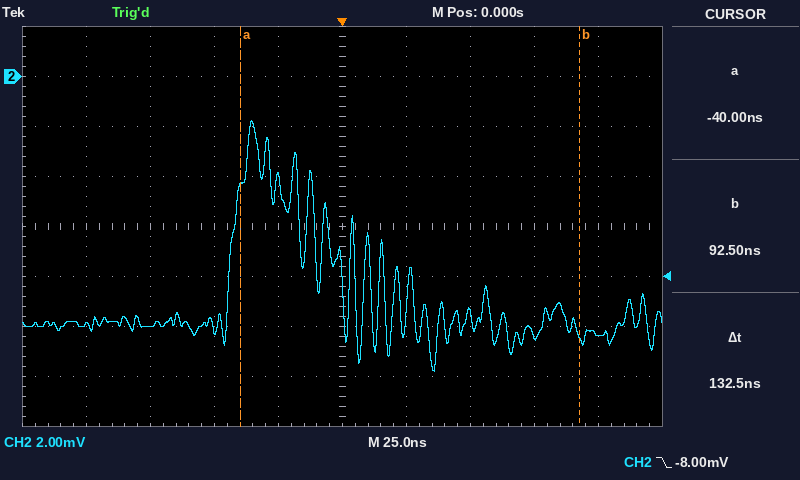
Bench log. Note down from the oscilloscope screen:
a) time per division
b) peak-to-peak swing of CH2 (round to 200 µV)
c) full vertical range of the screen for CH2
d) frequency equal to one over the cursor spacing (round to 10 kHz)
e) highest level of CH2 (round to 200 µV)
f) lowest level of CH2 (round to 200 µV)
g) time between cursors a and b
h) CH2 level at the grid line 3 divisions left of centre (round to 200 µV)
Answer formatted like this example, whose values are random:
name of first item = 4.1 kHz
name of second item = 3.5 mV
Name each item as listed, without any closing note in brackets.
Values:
time per division = 25 ns
peak-to-peak swing of CH2 = 10.0 mV
full vertical range of the screen for CH2 = 16 mV
frequency equal to one over the cursor spacing = 7.55 MHz
highest level of CH2 = -1.8 mV
lowest level of CH2 = -11.8 mV
time between cursors a and b = 132.5 ns
CH2 level at the grid line 3 divisions left of centre = -10.0 mV
